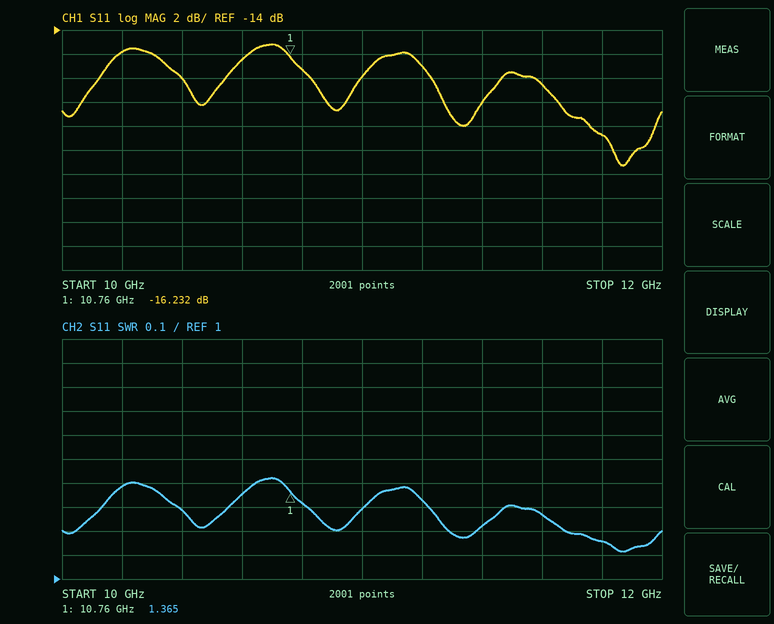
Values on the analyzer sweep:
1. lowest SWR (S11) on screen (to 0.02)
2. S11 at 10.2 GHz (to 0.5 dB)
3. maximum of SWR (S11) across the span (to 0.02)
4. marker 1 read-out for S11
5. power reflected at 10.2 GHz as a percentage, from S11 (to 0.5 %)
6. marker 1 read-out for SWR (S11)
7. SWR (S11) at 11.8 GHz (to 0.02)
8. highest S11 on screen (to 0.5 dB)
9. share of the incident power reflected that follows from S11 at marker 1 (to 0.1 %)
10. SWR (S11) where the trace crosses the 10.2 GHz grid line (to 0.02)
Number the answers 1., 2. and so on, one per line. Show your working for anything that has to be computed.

1. 1.12
2. -16.0 dB
3. 1.42
4. -16.232 dB
5. 10^(-16/10) ≈ 2.5 %
6. 1.365
7. 1.16
8. -15.0 dB
9. 10^(-16.232/10) ≈ 2.4 %
10. 1.38
